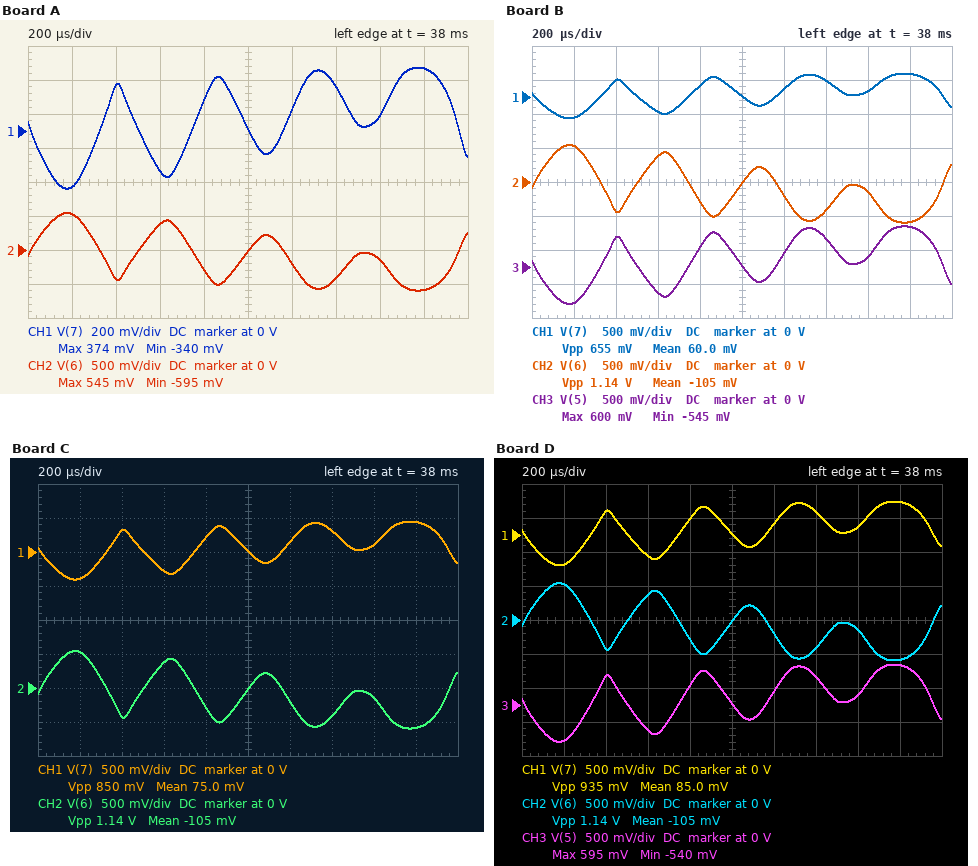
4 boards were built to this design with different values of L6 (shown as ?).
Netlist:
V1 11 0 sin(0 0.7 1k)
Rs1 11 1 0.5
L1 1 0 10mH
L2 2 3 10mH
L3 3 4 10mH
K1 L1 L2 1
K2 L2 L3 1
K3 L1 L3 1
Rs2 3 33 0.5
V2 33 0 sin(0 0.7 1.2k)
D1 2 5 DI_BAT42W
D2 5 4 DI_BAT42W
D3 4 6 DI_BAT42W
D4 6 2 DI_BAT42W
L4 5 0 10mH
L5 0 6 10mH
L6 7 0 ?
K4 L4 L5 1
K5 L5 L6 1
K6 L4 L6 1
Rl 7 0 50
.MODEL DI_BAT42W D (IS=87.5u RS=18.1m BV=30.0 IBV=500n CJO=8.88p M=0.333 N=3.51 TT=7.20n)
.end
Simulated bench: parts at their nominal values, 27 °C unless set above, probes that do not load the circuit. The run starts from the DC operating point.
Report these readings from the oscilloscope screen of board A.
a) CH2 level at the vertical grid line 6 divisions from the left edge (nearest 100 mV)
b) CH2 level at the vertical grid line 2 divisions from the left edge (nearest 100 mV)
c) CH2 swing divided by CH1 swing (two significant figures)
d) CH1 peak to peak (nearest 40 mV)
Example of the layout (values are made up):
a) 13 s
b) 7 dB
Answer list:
a) -200 mV
b) -400 mV
c) 1.6
d) 720 mV
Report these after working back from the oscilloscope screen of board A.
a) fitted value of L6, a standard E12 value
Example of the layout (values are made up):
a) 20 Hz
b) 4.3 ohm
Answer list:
a) 3.9 mH
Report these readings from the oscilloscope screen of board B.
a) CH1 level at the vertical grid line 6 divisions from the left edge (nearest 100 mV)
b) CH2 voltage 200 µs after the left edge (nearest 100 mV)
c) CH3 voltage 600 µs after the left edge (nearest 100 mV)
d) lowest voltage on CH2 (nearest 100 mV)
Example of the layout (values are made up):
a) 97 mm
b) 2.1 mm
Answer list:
a) 100 mV
b) 500 mV
c) -400 mV
d) -600 mV
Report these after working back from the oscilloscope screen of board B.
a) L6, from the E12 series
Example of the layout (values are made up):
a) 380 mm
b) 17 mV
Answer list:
a) 3.3 mH
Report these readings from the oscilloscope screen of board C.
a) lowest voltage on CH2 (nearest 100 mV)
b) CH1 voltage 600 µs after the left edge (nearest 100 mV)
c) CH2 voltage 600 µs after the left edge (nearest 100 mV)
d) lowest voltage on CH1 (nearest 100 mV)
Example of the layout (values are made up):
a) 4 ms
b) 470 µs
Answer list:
a) -600 mV
b) -300 mV
c) 400 mV
d) -400 mV
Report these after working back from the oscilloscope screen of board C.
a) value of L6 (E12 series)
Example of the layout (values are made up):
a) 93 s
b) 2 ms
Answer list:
a) 5.6 mH
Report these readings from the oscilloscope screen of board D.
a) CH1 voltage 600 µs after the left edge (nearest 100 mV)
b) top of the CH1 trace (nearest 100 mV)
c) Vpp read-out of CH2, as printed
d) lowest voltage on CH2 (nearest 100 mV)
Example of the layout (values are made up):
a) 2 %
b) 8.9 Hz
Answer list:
a) -300 mV
b) 500 mV
c) 1.14 V
d) -600 mV
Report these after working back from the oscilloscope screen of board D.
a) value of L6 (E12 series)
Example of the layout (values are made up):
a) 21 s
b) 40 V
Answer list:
a) 6.8 mH
